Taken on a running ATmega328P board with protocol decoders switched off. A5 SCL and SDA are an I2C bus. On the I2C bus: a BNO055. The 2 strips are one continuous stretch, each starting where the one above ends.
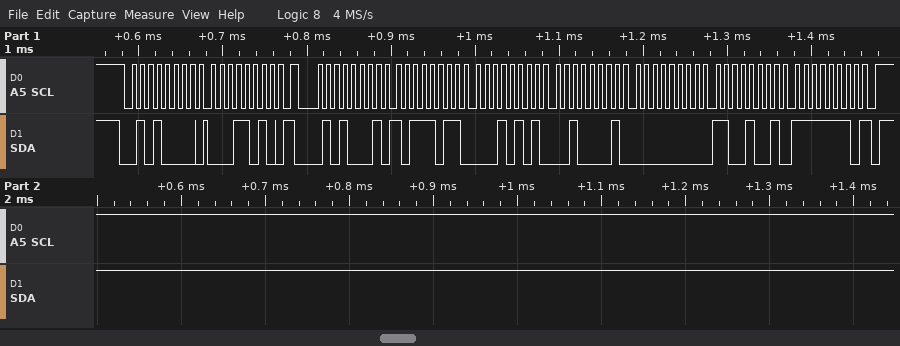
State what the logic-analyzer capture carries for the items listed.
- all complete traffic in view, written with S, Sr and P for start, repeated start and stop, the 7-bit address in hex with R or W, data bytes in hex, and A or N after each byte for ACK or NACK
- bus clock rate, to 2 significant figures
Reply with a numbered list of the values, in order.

1. S 28W A 1A A Sr 28R A BB A 15 A 21 A 00 A C9 A FE N P
2. 100 kHz
